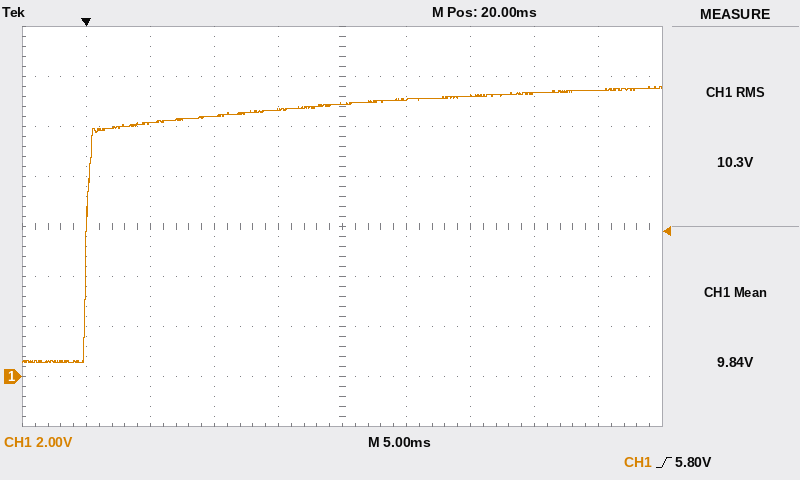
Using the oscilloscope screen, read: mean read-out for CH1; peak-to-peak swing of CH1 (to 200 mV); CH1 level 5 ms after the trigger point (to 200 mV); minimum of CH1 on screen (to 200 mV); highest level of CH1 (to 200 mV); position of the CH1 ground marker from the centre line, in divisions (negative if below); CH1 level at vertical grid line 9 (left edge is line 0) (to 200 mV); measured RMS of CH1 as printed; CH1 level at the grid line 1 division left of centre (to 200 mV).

9.84 V
11.0 V
10.2 V
600 mV
11.6 V
-3.0 div
11.4 V
10.3 V
10.6 V
